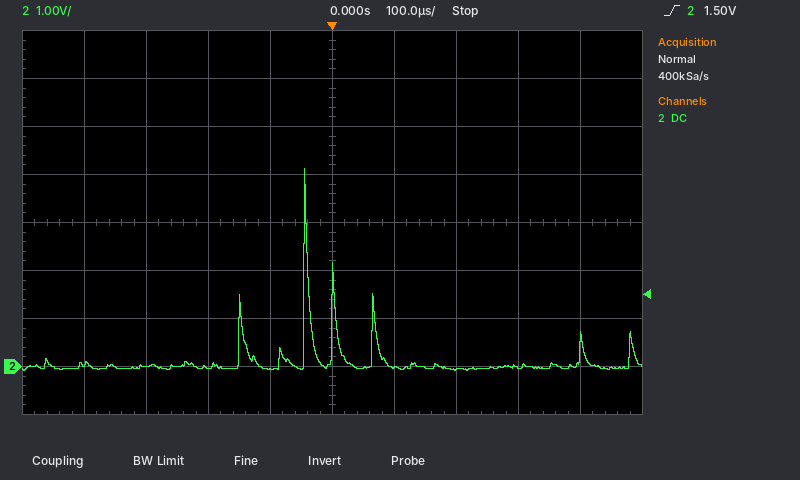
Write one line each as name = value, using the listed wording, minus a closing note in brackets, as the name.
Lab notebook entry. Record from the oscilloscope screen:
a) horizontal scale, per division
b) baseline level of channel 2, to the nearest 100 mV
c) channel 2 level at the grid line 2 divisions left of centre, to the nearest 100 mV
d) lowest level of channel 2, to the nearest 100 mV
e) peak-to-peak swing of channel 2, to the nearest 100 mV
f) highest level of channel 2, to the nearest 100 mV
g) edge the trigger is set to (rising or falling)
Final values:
horizontal scale, per division = 100 µs
baseline level of channel 2, to the nearest 100 mV = 0.0 V
channel 2 level at the grid line 2 divisions left of centre, to the nearest 100 mV = 0.0 V
lowest level of channel 2, to the nearest 100 mV = -100 mV
peak-to-peak swing of channel 2, to the nearest 100 mV = 4.2 V
highest level of channel 2, to the nearest 100 mV = 4.1 V
edge the trigger is set to = rising
